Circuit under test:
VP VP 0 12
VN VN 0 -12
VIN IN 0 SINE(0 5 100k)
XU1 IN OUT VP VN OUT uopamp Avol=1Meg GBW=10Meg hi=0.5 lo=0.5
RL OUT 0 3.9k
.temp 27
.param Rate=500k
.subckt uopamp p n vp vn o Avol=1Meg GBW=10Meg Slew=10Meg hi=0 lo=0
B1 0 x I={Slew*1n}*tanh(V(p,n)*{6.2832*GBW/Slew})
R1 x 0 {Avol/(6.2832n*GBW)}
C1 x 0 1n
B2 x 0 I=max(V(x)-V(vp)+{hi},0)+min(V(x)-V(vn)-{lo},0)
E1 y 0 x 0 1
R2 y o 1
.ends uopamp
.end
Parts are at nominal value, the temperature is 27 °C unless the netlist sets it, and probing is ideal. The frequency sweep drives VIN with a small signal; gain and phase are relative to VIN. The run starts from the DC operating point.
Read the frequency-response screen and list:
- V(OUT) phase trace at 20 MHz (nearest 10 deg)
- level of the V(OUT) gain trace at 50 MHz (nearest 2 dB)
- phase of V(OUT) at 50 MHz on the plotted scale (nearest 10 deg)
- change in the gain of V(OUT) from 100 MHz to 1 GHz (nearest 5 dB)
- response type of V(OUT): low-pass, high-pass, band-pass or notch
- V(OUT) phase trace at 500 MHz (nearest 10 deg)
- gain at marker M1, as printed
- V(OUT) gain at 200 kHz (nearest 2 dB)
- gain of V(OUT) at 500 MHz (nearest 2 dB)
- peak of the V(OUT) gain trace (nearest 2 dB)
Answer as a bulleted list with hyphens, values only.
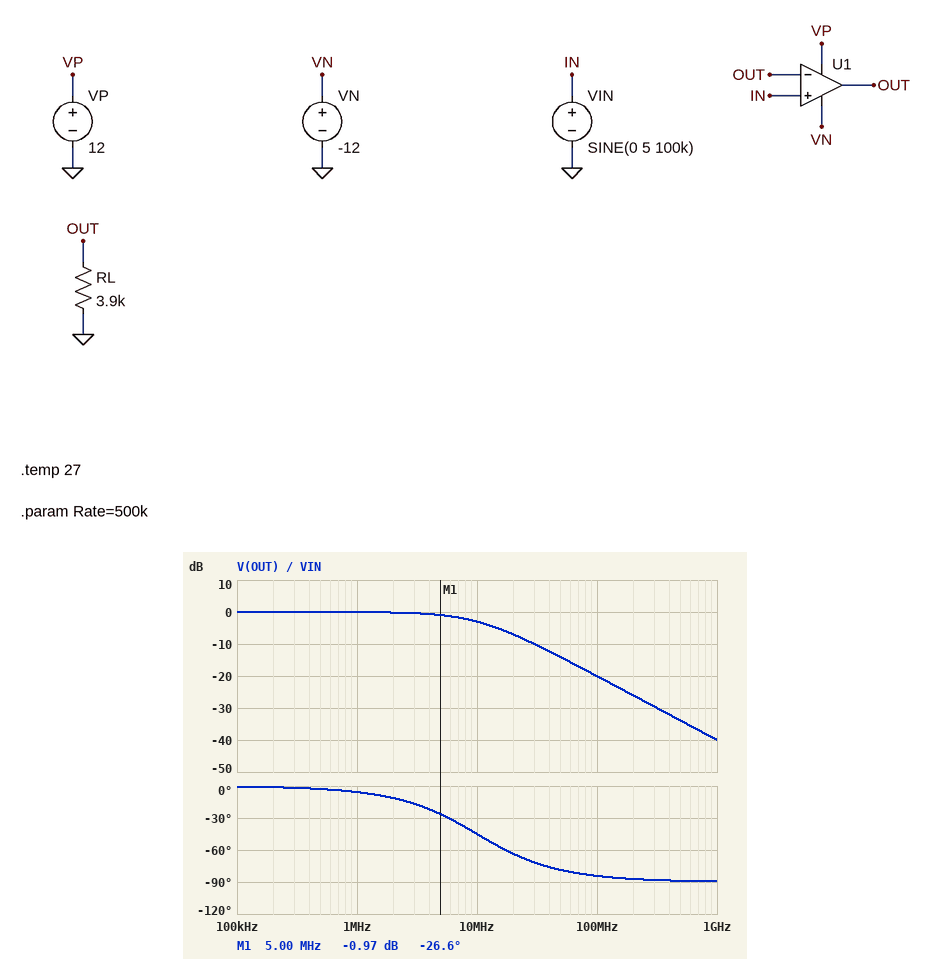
- -60 deg
- -14 dB
- -80 deg
- -20 dB
- low-pass
- -90 deg
- -0.97 dB
- 0 dB
- -34 dB
- 0 dB
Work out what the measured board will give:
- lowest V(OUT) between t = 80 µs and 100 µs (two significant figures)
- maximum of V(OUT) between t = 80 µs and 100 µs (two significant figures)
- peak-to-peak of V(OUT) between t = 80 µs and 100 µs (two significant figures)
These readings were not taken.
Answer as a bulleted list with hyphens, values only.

- -5.0 V
- 5.0 V
- 10 V
